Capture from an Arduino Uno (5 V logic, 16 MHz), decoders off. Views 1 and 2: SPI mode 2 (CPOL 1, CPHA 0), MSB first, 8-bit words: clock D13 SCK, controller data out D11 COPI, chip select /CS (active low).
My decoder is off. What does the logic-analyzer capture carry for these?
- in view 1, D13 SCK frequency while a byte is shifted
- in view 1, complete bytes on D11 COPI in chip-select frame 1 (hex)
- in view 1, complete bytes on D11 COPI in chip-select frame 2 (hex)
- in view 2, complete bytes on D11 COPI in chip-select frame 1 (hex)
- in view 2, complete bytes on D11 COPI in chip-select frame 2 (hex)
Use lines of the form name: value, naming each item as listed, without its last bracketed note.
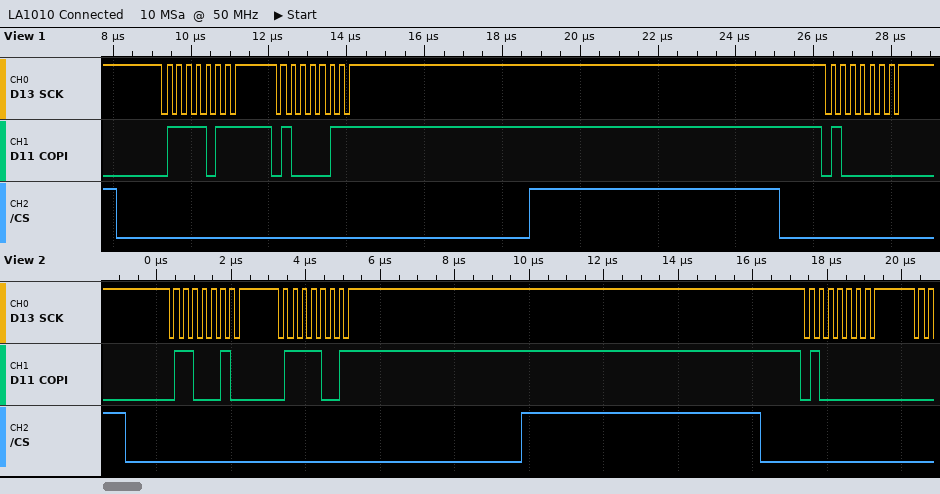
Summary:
in view 1, D13 SCK frequency while a byte is shifted: 4 MHz
in view 1, complete bytes on D11 COPI in chip-select frame 1: 0x7B 0x43
in view 1, complete bytes on D11 COPI in chip-select frame 2: 0x40
in view 2, complete bytes on D11 COPI in chip-select frame 1: 62 79
in view 2, complete bytes on D11 COPI in chip-select frame 2: 40
